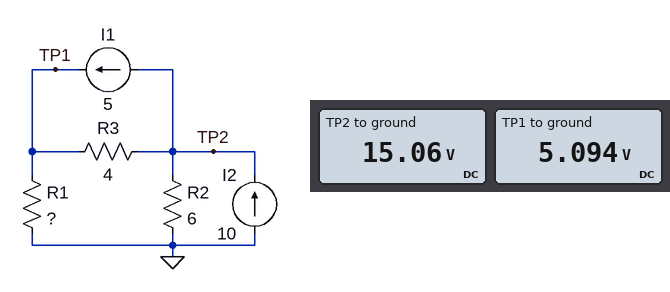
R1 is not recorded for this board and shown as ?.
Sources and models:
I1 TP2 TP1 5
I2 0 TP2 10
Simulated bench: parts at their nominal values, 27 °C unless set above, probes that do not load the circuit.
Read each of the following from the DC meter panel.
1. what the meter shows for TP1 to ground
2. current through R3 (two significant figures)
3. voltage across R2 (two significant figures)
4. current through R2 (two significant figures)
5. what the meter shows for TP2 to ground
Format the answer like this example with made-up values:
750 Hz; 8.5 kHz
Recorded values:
5.094 V; 2.5 A; 15 V; 2.5 A; 15.06 V
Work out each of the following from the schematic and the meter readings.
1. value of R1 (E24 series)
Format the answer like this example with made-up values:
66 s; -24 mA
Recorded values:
0.68 Ω
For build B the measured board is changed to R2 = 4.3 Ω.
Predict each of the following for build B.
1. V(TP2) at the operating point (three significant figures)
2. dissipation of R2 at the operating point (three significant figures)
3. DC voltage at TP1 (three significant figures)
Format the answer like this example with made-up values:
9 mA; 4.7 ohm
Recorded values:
12.8 V; 38.3 W; 4.77 V
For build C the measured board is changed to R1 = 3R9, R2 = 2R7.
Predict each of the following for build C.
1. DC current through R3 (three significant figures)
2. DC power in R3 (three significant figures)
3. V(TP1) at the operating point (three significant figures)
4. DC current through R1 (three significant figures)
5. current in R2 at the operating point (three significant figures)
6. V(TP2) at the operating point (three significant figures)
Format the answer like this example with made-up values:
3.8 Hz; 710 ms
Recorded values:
566 mA; 1.28 W; 17.3 V; 4.43 A; 5.57 A; 15.0 V
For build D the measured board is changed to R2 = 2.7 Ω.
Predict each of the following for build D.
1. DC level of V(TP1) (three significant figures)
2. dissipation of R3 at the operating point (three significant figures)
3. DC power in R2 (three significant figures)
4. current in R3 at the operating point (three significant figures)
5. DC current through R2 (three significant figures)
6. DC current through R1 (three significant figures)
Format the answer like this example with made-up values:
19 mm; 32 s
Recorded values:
4.33 V; 7.49 W; 35.6 W; 1.37 A; 3.63 A; 6.37 A
